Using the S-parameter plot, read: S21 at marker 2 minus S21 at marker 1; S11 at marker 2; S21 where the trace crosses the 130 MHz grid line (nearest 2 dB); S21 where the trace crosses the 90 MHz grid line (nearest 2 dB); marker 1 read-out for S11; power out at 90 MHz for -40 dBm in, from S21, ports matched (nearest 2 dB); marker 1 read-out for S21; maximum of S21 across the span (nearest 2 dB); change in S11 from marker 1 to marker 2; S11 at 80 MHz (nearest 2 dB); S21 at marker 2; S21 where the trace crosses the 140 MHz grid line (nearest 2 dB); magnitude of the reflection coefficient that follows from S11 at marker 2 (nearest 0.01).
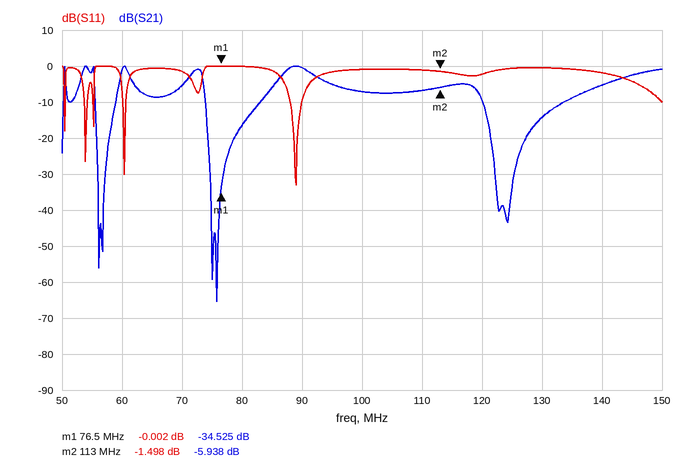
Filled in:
28.587 dB
-1.498 dB
-14 dB
0 dB
-0.002 dB
-40 dBm
-34.525 dB
0 dB
-1.496 dB
0 dB
-5.938 dB
-6 dB
0.84
